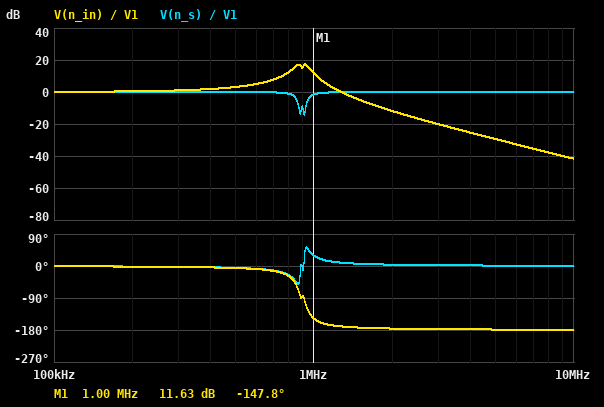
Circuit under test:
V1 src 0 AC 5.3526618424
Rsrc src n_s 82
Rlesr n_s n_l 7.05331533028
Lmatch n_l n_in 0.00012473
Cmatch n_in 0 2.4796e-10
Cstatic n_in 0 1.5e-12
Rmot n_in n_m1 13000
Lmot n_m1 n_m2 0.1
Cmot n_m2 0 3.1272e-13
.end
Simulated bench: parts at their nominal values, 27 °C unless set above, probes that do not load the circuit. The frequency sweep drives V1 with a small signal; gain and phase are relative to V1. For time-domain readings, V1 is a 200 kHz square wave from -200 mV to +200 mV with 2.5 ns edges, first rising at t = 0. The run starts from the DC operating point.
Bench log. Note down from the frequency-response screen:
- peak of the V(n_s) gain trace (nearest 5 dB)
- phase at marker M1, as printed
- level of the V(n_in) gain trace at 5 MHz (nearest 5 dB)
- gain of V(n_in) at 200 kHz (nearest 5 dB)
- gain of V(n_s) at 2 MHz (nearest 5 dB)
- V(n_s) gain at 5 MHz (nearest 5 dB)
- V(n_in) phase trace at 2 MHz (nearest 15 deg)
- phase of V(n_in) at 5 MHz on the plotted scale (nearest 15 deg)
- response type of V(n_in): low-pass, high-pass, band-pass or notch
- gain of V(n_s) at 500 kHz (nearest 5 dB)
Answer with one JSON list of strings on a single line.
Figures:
["0 dB", "-147.8 deg", "-30 dB", "0 dB", "0 dB", "0 dB", "-180 deg", "-180 deg", "low-pass", "0 dB"]
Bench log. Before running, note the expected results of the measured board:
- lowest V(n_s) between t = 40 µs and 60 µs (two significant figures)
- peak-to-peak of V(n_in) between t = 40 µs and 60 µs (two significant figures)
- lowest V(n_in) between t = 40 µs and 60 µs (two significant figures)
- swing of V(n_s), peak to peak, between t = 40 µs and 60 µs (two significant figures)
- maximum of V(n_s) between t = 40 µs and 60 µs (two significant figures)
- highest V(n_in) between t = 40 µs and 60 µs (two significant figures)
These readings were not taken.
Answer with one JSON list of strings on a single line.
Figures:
["-230 mV", "1.0 V", "-500 mV", "460 mV", "230 mV", "500 mV"]
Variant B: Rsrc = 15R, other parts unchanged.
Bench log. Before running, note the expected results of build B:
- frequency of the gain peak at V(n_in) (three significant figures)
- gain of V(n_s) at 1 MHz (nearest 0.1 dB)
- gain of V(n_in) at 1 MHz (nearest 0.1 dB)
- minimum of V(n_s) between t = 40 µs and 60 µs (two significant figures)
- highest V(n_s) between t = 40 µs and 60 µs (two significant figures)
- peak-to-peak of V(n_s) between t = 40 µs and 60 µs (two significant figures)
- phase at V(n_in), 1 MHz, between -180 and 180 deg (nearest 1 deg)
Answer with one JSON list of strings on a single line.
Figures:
["919 kHz", "-0.1 dB", "13.0 dB", "-210 mV", "210 mV", "410 mV", "-171 deg"]
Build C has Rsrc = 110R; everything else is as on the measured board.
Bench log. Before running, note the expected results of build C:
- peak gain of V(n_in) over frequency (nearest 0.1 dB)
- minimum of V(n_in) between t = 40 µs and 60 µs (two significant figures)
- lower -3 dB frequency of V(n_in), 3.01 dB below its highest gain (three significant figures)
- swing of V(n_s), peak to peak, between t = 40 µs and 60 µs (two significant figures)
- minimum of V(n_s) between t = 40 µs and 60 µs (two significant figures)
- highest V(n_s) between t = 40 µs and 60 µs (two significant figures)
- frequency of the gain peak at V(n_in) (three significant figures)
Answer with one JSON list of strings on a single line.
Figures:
["15.1 dB", "-490 mV", "805 kHz", "480 mV", "-240 mV", "240 mV", "873 kHz"]
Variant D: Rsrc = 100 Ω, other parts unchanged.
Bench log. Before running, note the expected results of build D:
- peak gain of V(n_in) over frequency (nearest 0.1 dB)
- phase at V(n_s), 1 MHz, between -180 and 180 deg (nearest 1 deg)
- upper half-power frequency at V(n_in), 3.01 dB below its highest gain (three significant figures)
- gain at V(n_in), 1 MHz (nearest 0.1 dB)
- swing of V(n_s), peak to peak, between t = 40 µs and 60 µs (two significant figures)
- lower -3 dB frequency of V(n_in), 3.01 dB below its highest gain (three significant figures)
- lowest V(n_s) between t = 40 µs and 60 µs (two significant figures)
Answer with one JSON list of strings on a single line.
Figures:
["15.8 dB", "34 deg", "976 kHz", "11.1 dB", "470 mV", "812 kHz", "-240 mV"]
